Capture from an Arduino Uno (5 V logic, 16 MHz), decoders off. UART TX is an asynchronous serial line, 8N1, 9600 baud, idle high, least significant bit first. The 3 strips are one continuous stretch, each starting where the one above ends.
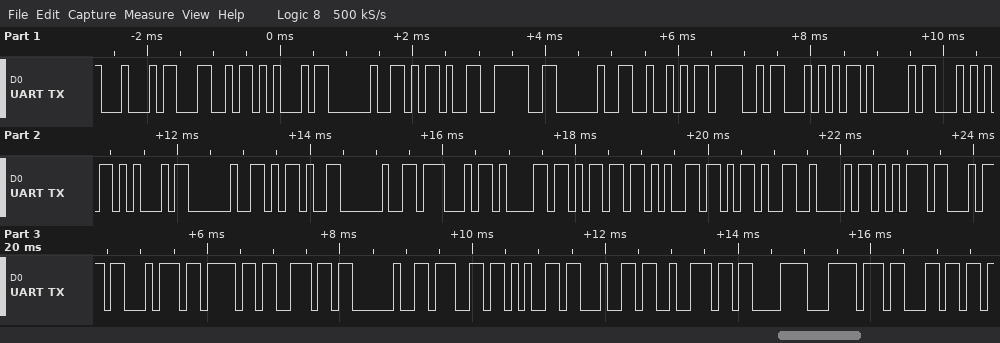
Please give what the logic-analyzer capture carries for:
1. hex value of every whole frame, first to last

44 4C 45 20 2D 3E 20 52 4F 54 41 54 45 20 2D 20 47 61 6D 65 2D 42 75 74 74 6F 6E 20 67 65 64 72 C3 BC 63
